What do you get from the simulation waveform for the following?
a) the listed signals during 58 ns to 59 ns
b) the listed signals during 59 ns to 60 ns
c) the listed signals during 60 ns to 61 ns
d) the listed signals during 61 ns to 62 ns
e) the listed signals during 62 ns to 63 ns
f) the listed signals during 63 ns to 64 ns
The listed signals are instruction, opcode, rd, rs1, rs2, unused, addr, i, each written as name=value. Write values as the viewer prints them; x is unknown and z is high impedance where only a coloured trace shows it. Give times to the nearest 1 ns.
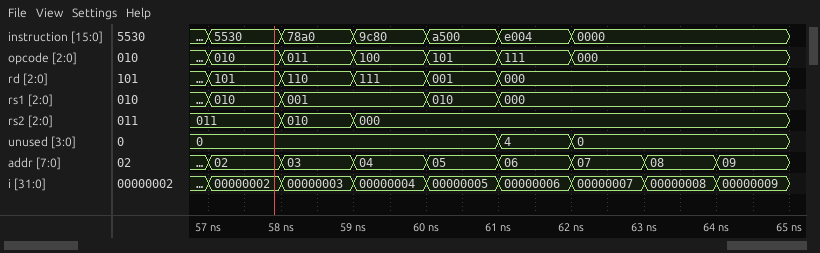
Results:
instruction=78a0, opcode=011, rd=110, rs1=001, rs2=010, unused=0, addr=03, i=00000003
instruction=9c80, opcode=100, rd=111, rs1=001, rs2=000, unused=0, addr=04, i=00000004
instruction=a500, opcode=101, rd=001, rs1=010, rs2=000, unused=0, addr=05, i=00000005
instruction=e004, opcode=111, rd=000, rs1=000, rs2=000, unused=4, addr=06, i=00000006
instruction=0000, opcode=000, rd=000, rs1=000, rs2=000, unused=0, addr=07, i=00000007
instruction=0000, opcode=000, rd=000, rs1=000, rs2=000, unused=0, addr=08, i=00000008
